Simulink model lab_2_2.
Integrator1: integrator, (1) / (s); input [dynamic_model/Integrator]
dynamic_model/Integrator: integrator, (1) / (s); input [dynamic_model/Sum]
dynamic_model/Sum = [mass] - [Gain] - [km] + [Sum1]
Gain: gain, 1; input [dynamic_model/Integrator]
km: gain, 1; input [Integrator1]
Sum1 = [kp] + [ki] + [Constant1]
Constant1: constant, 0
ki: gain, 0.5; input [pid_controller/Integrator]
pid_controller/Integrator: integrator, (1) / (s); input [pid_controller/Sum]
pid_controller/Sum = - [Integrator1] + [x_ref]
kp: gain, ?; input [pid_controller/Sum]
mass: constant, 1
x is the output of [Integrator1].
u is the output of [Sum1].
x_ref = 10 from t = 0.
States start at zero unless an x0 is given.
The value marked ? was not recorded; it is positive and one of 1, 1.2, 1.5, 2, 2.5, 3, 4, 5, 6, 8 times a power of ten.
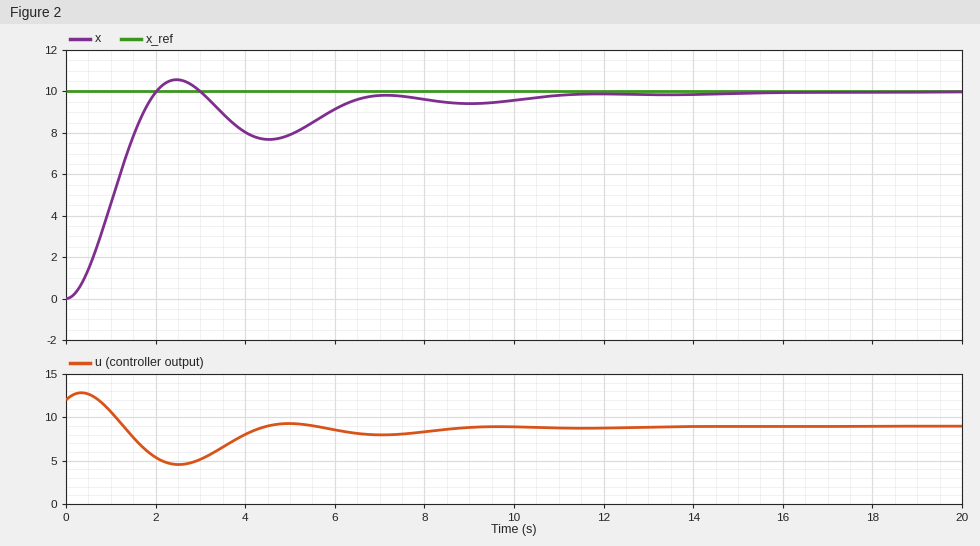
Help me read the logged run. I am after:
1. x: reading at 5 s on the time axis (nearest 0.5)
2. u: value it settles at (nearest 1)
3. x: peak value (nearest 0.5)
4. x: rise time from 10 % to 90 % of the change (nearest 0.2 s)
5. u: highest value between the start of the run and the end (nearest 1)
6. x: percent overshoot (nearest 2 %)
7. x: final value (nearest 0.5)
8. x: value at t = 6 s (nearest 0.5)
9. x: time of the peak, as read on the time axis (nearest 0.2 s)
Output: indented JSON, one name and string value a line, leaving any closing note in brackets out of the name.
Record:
{
  "x: reading at 5 s on the time axis": "8.0",
  "u: value it settles at": "9",
  "x: peak value": "10.5",
  "x: rise time from 10 % to 90 % of the change": "1.4 s",
  "u: highest value between the start of the run and the end": "13",
  "x: percent overshoot": "6 %",
  "x: final value": "10.0",
  "x: value at t = 6 s": "9.0",
  "x: time of the peak, as read on the time axis": "2.4 s"
}
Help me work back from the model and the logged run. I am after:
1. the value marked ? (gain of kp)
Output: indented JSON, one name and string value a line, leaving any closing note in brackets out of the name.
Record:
{
  "the value marked ?": "1.2"
}
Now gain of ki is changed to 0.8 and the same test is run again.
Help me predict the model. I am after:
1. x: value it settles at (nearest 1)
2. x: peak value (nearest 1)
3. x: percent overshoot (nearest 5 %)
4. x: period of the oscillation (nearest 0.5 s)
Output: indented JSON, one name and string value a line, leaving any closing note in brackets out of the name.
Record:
{
  "x: value it settles at": "10",
  "x: peak value": "12",
  "x: percent overshoot": "20 %",
  "x: period of the oscillation": "4.5 s"
}
